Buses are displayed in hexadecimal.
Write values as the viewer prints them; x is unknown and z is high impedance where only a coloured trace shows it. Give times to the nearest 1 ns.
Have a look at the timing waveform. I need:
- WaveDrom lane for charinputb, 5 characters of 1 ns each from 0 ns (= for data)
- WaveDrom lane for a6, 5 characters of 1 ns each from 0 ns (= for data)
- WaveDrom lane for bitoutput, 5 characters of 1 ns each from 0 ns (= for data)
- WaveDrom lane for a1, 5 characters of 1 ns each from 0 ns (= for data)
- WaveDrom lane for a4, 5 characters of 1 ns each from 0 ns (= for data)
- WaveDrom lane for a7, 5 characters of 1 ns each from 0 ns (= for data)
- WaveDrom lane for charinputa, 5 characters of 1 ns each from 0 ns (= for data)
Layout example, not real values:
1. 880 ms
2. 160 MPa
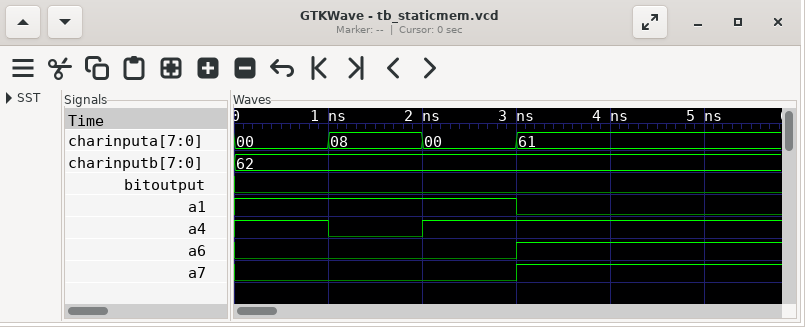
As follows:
1. {name: 'charinputb', wave: '=....', data: '62'}
2. {name: 'a6', wave: '0..1.'}
3. {name: 'bitoutput', wave: '0....'}
4. {name: 'a1', wave: '1..0.'}
5. {name: 'a4', wave: '101..'}
6. {name: 'a7', wave: '0..1.'}
7. {name: 'charinputa', wave: '====.', data: '00 08 00 61'}
